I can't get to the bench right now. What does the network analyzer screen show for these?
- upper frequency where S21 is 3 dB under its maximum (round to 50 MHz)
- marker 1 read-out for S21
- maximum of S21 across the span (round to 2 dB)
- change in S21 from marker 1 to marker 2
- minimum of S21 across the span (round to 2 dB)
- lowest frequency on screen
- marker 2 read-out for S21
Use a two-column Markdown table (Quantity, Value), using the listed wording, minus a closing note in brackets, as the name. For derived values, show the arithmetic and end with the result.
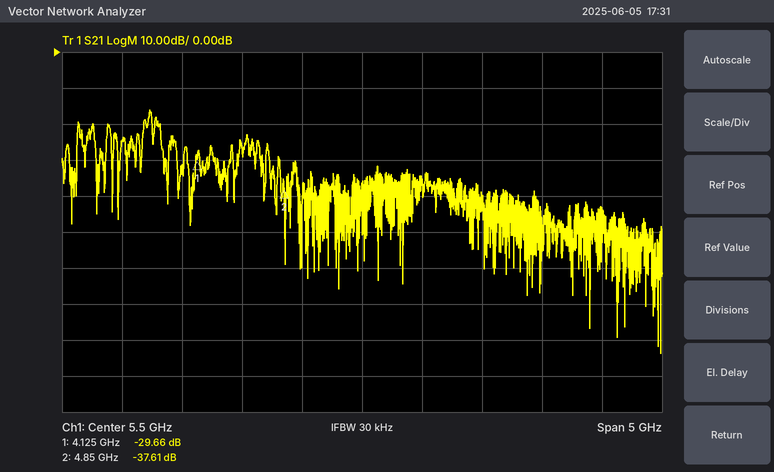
| Quantity | Value |
|---|---|
| upper frequency where S21 is 3 dB under its maximum | 3.75 GHz |
| marker 1 read-out for S21 | -29.66 dB |
| maximum of S21 across the span | -16 dB |
| change in S21 from marker 1 to marker 2 | -37.61 − (-29.66) = -7.95 dB |
| minimum of S21 across the span | -84 dB |
| lowest frequency on screen | 3 GHz |
| marker 2 read-out for S21 | -37.61 dB |
